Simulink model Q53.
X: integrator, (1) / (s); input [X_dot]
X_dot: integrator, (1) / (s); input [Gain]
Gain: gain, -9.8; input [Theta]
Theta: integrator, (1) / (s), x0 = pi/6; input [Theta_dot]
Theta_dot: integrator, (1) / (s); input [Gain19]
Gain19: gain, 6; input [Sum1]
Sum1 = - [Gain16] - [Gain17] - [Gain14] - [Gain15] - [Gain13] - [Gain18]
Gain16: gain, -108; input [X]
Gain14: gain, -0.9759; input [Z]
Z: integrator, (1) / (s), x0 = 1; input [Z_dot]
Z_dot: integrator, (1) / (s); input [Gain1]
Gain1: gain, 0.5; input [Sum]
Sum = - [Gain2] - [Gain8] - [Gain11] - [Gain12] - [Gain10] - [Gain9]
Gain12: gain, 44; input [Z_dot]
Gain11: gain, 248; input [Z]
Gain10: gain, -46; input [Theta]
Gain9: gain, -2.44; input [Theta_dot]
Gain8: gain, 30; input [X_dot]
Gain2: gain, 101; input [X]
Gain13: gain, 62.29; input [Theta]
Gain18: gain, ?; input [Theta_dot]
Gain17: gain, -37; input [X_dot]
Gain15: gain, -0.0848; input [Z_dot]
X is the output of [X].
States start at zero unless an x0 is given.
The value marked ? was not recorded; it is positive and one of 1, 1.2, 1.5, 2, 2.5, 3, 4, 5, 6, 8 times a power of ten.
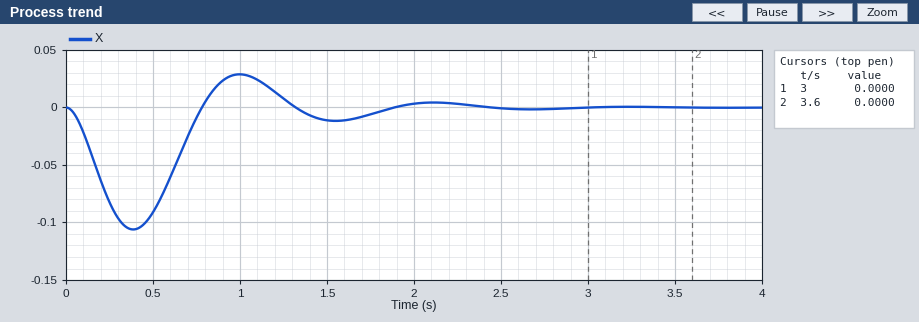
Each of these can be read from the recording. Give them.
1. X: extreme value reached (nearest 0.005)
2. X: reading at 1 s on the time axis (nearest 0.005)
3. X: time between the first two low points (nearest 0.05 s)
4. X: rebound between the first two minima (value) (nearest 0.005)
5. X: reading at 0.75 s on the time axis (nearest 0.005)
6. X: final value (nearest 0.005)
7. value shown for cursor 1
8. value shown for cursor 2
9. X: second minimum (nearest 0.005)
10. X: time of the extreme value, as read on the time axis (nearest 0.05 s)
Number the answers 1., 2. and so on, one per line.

1. -0.105
2. 0.030
3. 1.15 s
4. 0.030
5. -0.010
6. 0.000
7. 0.0000
8. 0.0000
9. -0.010
10. 0.40 s
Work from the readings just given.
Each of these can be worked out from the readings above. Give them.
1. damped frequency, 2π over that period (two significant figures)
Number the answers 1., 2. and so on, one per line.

1. 5.5 rad/s
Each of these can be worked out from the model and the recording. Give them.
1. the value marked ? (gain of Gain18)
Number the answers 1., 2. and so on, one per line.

1. 8
